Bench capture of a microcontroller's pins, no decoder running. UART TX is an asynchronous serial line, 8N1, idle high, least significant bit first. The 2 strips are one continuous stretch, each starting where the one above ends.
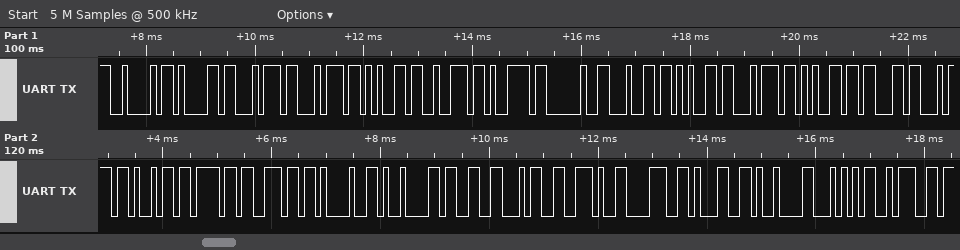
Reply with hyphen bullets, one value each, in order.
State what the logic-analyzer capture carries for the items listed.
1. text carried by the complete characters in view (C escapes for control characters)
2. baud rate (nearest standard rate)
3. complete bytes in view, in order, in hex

- "Battery detection!\t34.81\tT:"
- 9600 baud
- 42 61 74 74 65 72 79 20 64 65 74 65 63 74 69 6F 6E 21 09 33 34 2E 38 31 09 54 3A
